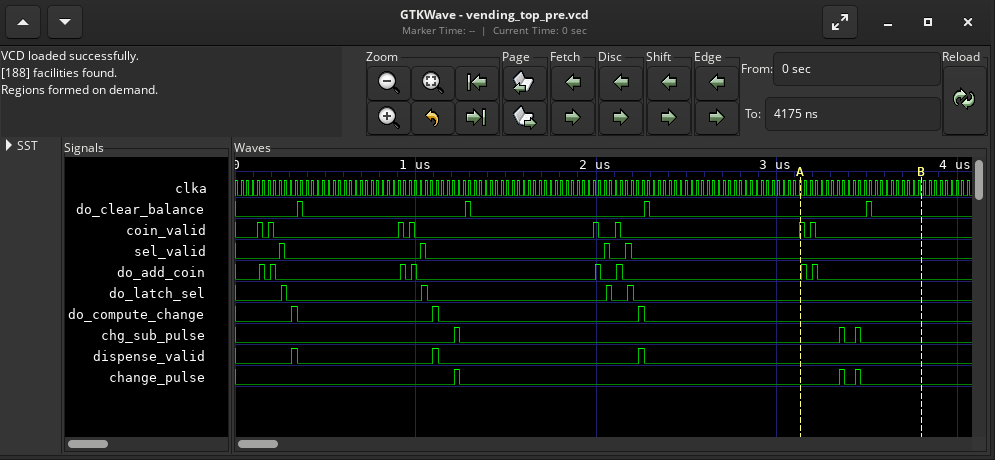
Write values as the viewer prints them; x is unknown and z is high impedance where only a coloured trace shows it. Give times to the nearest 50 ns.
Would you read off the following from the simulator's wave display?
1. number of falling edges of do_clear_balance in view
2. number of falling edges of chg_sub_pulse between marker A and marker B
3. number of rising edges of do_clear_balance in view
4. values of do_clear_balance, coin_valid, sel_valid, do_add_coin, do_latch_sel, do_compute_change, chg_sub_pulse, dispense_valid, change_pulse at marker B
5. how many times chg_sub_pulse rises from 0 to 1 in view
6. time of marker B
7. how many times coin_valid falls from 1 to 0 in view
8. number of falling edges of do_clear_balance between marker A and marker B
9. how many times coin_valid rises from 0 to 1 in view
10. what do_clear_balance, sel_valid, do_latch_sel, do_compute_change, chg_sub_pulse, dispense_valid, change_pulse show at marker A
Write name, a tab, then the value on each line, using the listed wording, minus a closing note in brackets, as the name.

number of falling edges of do_clear_balance in view	4
number of falling edges of chg_sub_pulse between marker A and marker B	2
number of rising edges of do_clear_balance in view	4
values of do_clear_balance, coin_valid, sel_valid, do_add_coin, do_latch_sel, do_compute_change, chg_sub_pulse, dispense_valid, change_pulse at marker B	do_clear_balance=0, coin_valid=0, sel_valid=0, do_add_coin=0, do_latch_sel=0, do_compute_change=0, chg_sub_pulse=0, dispense_valid=0, change_pulse=0
how many times chg_sub_pulse rises from 0 to 1 in view	3
time of marker B	3800 ns
how many times coin_valid falls from 1 to 0 in view	8
number of falling edges of do_clear_balance between marker A and marker B	1
how many times coin_valid rises from 0 to 1 in view	8
what do_clear_balance, sel_valid, do_latch_sel, do_compute_change, chg_sub_pulse, dispense_valid, change_pulse show at marker A	do_clear_balance=0, sel_valid=0, do_latch_sel=0, do_compute_change=0, chg_sub_pulse=0, dispense_valid=0, change_pulse=0
